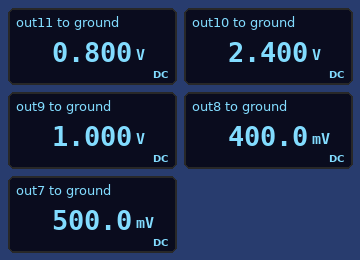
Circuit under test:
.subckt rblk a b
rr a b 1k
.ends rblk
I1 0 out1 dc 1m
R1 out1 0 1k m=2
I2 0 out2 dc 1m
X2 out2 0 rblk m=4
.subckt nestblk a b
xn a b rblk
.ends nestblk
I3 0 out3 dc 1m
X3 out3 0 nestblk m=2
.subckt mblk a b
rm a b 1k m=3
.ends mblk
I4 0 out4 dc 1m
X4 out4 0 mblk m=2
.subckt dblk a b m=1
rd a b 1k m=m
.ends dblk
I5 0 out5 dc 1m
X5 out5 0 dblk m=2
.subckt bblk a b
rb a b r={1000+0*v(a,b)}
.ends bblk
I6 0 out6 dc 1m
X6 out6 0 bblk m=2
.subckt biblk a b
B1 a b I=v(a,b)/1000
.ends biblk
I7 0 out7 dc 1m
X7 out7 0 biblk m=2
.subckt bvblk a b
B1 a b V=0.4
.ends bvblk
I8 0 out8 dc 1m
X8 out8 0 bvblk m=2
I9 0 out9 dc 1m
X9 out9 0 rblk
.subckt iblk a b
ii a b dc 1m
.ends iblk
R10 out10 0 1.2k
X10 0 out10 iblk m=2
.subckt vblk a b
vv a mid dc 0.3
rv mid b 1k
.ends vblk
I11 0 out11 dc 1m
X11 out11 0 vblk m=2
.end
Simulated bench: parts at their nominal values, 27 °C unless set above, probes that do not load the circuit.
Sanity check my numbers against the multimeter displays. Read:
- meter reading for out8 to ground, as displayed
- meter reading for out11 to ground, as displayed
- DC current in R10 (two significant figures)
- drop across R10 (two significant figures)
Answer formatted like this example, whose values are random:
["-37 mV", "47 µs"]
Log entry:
["400.0 mV", "0.800 V", "2.0 mA", "2.4 V"]
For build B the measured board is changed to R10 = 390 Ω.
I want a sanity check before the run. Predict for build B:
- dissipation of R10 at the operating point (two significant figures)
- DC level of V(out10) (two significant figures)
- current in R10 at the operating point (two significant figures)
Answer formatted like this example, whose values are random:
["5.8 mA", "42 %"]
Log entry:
["1.6 mW", "780 mV", "2.0 mA"]
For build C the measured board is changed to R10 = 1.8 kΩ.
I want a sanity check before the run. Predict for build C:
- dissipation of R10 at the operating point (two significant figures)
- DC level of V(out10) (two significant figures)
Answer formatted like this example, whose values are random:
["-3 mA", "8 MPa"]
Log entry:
["7.2 mW", "3.6 V"]
